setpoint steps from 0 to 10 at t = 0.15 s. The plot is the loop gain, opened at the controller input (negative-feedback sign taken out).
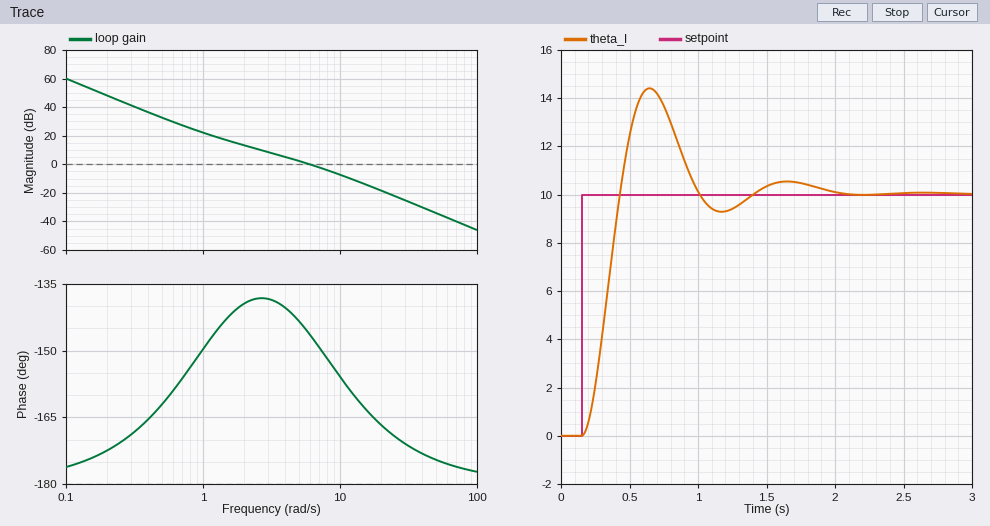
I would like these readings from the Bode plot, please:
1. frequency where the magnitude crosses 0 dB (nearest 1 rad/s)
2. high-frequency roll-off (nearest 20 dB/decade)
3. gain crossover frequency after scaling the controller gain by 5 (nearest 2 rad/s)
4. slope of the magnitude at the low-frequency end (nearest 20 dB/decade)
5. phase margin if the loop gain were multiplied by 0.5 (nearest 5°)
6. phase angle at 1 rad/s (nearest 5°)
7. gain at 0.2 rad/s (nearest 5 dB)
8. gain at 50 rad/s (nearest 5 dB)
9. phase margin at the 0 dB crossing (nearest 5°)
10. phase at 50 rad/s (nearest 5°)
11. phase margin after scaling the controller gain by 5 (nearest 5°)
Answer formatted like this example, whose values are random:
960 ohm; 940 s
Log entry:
6 rad/s; -40 dB/decade; 16 rad/s; -40 dB/decade; 40°; -150°; 50 dB; -35 dB; 35°; -175°; 15°
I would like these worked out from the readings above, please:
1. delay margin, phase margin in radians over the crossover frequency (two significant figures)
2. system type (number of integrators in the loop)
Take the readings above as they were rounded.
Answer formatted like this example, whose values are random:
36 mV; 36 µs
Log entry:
0.10 s; 2
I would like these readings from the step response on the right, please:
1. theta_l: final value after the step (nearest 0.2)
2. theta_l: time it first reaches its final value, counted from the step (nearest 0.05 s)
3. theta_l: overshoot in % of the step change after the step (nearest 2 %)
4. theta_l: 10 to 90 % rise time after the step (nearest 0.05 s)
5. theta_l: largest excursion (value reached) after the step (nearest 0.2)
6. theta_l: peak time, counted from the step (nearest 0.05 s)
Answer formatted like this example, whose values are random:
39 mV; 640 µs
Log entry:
10.0; 0.30 s; 44 %; 0.20 s; 14.4; 0.50 s
